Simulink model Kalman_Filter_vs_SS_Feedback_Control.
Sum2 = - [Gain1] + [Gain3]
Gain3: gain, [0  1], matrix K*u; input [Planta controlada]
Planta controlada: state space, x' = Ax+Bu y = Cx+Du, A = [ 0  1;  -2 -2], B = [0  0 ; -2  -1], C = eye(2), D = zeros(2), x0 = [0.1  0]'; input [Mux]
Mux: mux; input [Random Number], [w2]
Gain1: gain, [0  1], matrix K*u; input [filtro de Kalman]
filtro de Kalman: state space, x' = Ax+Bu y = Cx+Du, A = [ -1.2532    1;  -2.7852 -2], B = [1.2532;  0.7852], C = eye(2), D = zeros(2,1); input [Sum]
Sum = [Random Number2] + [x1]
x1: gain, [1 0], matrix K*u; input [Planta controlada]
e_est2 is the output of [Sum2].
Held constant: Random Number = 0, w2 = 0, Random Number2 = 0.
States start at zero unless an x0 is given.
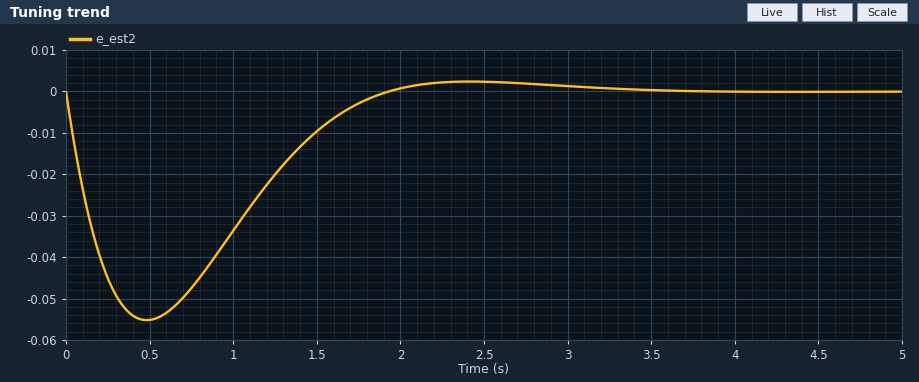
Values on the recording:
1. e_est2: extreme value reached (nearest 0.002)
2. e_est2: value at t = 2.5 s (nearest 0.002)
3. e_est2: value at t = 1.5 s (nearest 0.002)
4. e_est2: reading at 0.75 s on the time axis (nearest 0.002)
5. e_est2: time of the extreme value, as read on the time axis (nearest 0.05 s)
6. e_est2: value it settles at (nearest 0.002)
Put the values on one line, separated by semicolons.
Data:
-0.056; 0.002; -0.010; -0.048; 0.50 s; 0.000
